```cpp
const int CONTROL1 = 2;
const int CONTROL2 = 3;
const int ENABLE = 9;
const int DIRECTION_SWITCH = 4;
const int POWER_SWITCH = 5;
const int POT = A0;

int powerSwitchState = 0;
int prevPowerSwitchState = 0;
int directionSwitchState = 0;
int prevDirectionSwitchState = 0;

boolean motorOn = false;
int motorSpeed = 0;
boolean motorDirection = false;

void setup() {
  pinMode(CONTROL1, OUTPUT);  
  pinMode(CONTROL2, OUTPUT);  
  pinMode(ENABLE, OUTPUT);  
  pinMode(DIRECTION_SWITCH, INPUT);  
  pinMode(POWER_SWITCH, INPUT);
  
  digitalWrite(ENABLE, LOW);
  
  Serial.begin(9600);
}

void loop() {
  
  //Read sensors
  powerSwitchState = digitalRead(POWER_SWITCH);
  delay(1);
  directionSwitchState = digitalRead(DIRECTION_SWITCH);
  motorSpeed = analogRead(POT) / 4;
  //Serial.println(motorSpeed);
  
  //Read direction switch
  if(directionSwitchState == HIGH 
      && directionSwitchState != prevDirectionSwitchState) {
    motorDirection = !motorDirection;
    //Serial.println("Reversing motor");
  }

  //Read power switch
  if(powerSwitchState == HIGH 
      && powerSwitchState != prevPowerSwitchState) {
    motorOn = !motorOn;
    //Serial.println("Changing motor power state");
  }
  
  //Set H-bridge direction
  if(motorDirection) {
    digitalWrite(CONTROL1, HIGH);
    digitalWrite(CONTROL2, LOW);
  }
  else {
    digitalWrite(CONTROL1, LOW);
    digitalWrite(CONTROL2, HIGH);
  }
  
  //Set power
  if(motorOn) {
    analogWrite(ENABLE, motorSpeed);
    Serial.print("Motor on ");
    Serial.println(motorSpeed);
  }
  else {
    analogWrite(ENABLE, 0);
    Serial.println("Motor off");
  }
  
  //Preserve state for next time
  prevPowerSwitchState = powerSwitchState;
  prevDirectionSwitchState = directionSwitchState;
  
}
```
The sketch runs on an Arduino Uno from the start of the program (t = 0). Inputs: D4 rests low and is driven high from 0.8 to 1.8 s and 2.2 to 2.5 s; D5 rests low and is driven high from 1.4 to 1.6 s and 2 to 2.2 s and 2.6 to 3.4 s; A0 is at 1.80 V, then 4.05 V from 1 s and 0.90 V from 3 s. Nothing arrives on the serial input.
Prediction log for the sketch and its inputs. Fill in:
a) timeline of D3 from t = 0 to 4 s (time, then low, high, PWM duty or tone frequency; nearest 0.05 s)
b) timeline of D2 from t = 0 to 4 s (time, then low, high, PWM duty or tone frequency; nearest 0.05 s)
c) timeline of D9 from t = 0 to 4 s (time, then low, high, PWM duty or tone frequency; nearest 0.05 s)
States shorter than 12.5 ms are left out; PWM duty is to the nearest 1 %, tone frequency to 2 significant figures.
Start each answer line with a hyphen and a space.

- 0 s high; 0.8 s low; 2.2 s high
- 0 s low; 0.8 s high; 2.2 s low
- 0 s low; 1.4 s PWM 81 %; 2 s low; 2.6 s PWM 81 %; 3 s PWM 18 %
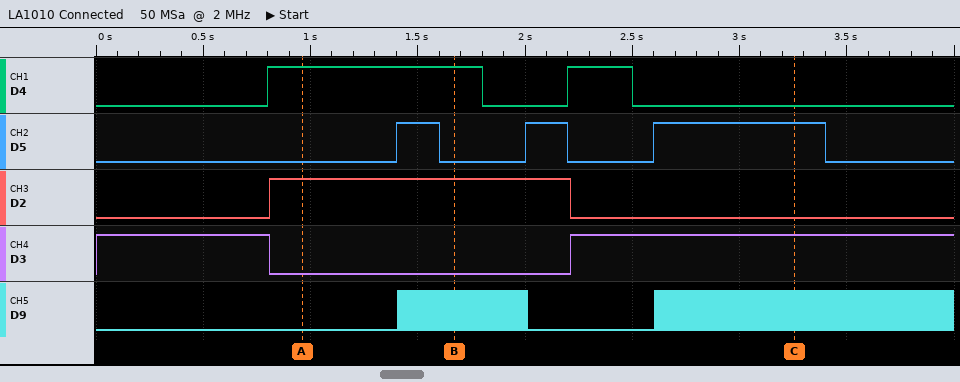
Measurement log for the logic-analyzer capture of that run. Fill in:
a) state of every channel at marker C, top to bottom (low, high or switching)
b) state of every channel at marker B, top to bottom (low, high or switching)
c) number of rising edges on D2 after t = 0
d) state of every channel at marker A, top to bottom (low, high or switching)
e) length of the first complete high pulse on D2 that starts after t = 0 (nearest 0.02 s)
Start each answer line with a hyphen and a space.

- D4 low, D5 high, D2 low, D3 high, D9 switching
- D4 high, D5 low, D2 high, D3 low, D9 switching
- 1
- D4 high, D5 low, D2 high, D3 low, D9 low
- 1.40 s
